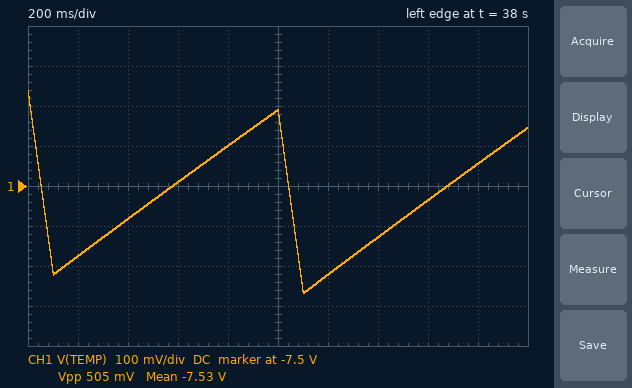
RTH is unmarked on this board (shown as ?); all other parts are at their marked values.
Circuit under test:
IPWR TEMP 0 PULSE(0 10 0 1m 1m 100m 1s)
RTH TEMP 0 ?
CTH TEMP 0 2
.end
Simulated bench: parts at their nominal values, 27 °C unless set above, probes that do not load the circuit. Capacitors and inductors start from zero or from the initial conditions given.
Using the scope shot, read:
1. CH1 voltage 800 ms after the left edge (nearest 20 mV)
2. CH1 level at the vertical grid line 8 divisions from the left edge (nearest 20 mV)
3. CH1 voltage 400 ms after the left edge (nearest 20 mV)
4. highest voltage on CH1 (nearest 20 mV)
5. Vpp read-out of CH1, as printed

-7.40 V
-7.54 V
-7.58 V
-7.26 V
505 mV
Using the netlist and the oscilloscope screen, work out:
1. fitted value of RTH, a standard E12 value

8.2 Ω
